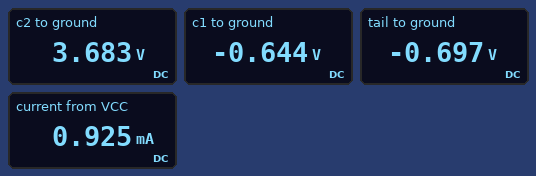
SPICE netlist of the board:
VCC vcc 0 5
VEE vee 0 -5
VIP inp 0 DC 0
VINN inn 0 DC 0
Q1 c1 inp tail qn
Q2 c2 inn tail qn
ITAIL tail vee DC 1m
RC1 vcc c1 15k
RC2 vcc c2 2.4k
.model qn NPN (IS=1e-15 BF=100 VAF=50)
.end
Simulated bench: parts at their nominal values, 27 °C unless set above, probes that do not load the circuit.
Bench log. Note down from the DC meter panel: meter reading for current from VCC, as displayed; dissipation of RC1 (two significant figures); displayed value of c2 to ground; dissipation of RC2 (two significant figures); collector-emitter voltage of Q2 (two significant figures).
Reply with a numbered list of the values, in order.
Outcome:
1. 0.925 mA
2. 2.1 mW
3. 3.683 V
4. 720 µW
5. 4.4 V
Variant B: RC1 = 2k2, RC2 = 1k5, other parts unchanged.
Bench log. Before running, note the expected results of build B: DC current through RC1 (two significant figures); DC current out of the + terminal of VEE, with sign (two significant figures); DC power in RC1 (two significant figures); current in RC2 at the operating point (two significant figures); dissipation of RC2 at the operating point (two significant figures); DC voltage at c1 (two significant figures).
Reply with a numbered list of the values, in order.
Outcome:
1. 490 µA
2. -1.0 mA
3. 540 µW
4. 500 µA
5. 370 µW
6. 3.9 V
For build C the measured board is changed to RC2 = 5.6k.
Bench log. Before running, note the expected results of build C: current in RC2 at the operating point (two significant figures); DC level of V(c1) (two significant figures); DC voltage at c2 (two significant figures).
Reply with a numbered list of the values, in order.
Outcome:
1. 540 µA
2. -650 mV
3. 2.0 V
